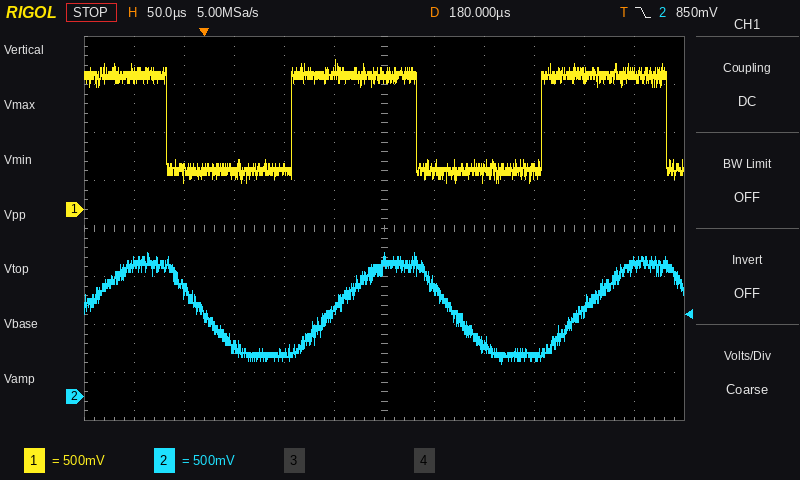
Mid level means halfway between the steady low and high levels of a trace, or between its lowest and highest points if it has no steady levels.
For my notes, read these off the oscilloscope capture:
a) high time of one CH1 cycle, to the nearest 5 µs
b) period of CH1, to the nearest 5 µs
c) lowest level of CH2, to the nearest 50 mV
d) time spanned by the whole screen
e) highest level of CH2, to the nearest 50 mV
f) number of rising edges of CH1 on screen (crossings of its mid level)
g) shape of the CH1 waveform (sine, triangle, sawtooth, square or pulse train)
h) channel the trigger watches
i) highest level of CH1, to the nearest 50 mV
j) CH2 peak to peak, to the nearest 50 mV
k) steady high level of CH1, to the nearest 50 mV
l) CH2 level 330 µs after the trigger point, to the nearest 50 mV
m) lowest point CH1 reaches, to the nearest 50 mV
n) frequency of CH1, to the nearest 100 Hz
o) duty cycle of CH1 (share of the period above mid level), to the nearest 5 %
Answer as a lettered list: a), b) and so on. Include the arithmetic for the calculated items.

a) 125 µs
b) 250 µs
c) 350 mV
d) 600 µs
e) 1.50 V
f) 2
g) square
h) CH2
i) 1.55 V
j) 1.50 V − (350 mV) = 1.15 V
k) 1.40 V
l) 400 mV
m) 300 mV
n) 1 / 250 µs ≈ 4.0 kHz
o) 125 µs / 250 µs ≈ 50 %
